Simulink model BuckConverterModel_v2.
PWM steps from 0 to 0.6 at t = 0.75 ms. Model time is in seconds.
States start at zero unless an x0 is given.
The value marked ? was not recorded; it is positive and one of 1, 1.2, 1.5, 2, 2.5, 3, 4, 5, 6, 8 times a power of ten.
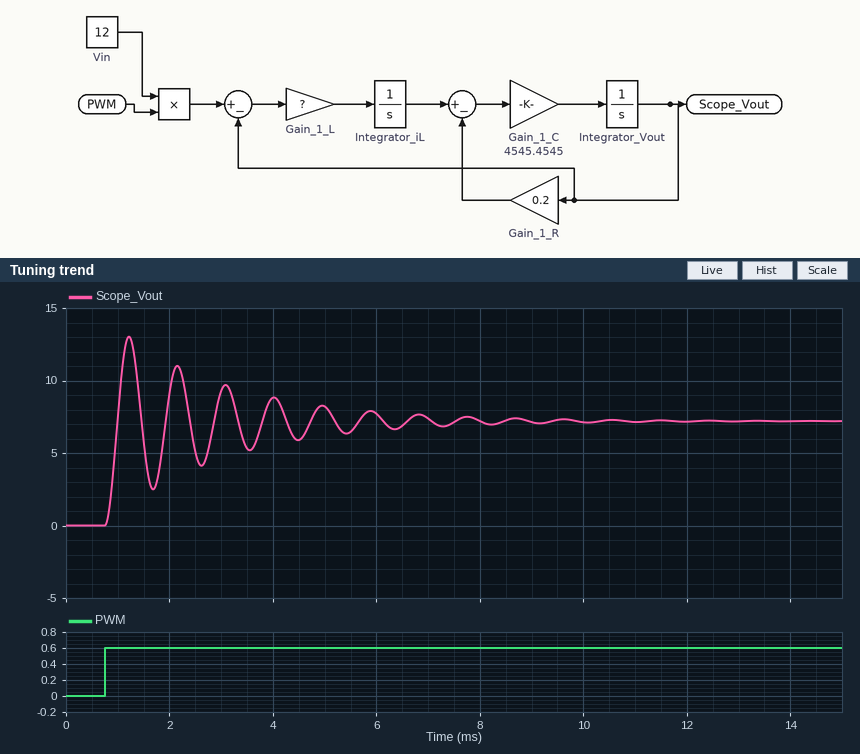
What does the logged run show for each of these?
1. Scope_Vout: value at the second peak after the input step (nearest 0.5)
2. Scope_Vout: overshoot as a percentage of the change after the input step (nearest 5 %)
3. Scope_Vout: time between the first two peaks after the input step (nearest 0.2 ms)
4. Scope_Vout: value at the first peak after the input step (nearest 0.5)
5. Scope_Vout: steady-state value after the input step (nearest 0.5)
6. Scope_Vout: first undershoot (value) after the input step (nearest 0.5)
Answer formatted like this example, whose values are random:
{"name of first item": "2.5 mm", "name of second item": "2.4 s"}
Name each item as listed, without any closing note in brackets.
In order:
{"Scope_Vout: value at the second peak after the input step": "11.0", "Scope_Vout: overshoot as a percentage of the change after the input step": "80 %", "Scope_Vout: time between the first two peaks after the input step": "1.0 ms", "Scope_Vout: value at the first peak after the input step": "13.0", "Scope_Vout: steady-state value after the input step": "7.0", "Scope_Vout: first undershoot (value) after the input step": "2.5"}
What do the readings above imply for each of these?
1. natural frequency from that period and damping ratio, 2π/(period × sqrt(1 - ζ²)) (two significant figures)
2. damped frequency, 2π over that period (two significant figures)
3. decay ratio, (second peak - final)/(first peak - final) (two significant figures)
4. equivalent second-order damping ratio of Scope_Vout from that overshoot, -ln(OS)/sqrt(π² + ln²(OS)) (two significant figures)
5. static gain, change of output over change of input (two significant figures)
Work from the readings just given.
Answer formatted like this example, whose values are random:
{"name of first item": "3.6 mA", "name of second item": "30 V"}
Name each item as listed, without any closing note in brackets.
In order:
{"natural frequency from that period and damping ratio, 2π/(period × sqrt(1 - ζ²))": "6.3 rad/ms", "damped frequency, 2π over that period": "6.3 rad/ms", "decay ratio, (second peak - final)/(first peak - final)": "0.67", "equivalent second-order damping ratio of Scope_Vout from that overshoot, -ln(OS)/sqrt(π² + ln²(OS))": "0.071", "static gain, change of output over change of input": "12"}
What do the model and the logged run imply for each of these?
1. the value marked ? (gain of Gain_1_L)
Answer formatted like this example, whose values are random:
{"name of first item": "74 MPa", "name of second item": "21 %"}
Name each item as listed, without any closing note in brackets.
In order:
{"the value marked ?": "10000"}
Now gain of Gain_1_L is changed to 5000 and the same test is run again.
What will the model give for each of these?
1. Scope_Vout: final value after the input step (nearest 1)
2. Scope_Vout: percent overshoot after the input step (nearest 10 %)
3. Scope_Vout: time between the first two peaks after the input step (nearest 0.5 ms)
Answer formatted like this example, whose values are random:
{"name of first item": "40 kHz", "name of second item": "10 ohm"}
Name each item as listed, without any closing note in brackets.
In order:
{"Scope_Vout: final value after the input step": "7", "Scope_Vout: percent overshoot after the input step": "70 %", "Scope_Vout: time between the first two peaks after the input step": "1.5 ms"}
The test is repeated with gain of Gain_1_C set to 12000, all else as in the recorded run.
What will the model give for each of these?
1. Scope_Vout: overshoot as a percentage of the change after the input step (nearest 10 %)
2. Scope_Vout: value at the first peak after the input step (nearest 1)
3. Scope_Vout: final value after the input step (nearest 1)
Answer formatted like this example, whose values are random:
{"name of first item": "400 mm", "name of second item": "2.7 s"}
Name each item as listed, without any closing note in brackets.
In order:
{"Scope_Vout: overshoot as a percentage of the change after the input step": "70 %", "Scope_Vout: value at the first peak after the input step": "12", "Scope_Vout: final value after the input step": "7"}
